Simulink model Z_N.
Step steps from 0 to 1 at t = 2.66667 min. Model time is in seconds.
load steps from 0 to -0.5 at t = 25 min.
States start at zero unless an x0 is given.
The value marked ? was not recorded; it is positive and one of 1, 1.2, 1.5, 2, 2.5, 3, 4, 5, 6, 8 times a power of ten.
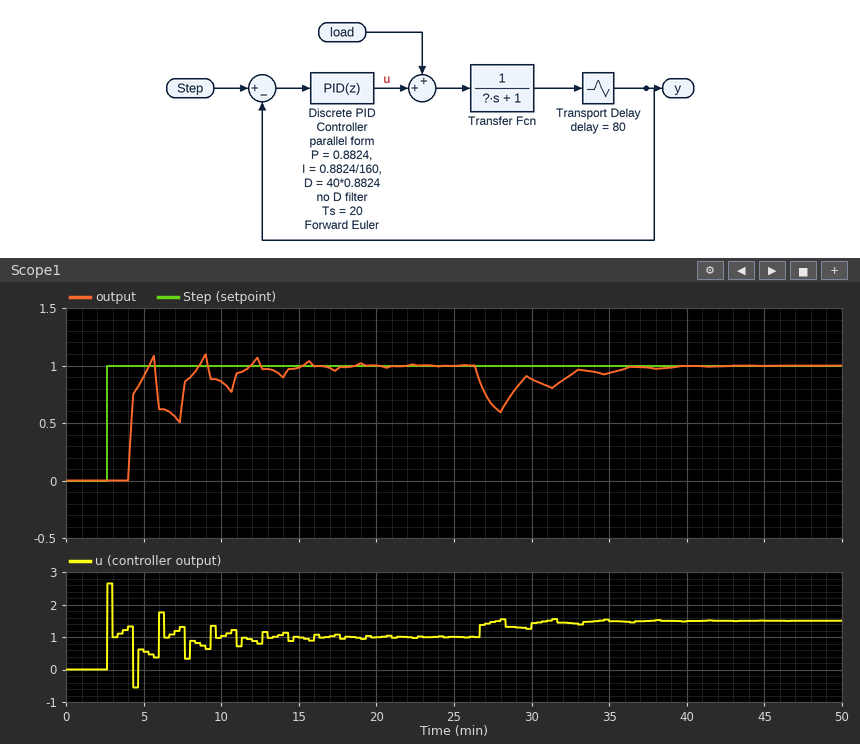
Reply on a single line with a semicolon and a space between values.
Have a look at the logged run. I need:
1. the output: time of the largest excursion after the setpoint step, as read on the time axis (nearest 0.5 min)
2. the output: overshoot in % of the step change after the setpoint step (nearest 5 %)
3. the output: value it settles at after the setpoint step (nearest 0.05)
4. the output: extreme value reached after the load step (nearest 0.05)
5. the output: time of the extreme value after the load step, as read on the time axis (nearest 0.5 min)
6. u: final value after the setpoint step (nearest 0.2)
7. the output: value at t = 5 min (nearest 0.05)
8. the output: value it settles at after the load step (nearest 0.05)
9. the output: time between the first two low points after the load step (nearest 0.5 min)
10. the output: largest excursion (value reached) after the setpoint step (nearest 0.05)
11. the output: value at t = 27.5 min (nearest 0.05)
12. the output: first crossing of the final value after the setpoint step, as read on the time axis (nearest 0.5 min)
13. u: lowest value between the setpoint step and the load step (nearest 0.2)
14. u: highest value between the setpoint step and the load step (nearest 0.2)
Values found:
9.0 min; 10 %; 1.00; 0.60; 28.0 min; 1.0; 0.90; 1.00; 3.5 min; 1.10; 0.65; 5.5 min; -0.6; 2.6
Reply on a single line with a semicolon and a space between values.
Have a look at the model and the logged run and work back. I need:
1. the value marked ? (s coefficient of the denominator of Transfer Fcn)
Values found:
60
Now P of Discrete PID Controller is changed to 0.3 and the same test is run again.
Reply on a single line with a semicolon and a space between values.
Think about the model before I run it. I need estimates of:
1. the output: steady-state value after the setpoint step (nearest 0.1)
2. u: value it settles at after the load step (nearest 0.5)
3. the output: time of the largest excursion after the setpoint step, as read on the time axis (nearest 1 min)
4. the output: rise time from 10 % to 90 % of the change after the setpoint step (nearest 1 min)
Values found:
1.0; 1.5; 11 min; 5 min
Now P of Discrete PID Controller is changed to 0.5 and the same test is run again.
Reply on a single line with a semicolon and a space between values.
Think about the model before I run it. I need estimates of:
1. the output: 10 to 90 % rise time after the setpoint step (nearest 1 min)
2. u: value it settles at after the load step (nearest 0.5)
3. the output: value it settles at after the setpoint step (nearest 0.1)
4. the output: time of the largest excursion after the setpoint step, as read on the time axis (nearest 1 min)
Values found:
4 min; 1.5; 1.0; 11 min
